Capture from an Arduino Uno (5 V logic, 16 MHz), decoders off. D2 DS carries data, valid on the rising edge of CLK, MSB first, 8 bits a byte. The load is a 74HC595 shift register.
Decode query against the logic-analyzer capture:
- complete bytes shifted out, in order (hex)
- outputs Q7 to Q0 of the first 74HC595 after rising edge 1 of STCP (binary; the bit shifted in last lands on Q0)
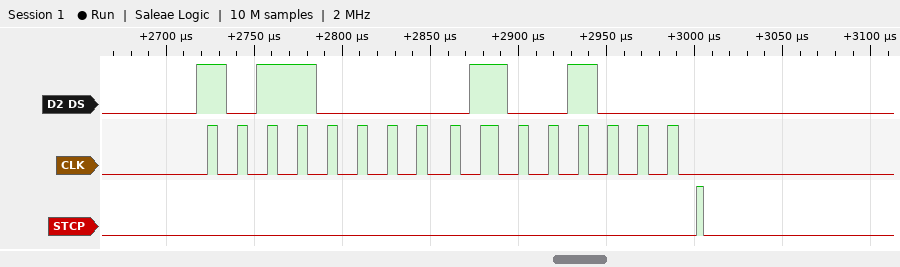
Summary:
B0 48
01001000
